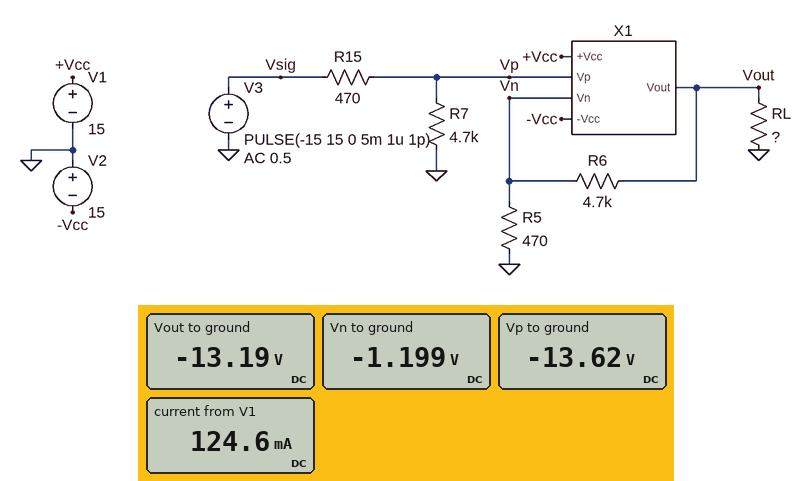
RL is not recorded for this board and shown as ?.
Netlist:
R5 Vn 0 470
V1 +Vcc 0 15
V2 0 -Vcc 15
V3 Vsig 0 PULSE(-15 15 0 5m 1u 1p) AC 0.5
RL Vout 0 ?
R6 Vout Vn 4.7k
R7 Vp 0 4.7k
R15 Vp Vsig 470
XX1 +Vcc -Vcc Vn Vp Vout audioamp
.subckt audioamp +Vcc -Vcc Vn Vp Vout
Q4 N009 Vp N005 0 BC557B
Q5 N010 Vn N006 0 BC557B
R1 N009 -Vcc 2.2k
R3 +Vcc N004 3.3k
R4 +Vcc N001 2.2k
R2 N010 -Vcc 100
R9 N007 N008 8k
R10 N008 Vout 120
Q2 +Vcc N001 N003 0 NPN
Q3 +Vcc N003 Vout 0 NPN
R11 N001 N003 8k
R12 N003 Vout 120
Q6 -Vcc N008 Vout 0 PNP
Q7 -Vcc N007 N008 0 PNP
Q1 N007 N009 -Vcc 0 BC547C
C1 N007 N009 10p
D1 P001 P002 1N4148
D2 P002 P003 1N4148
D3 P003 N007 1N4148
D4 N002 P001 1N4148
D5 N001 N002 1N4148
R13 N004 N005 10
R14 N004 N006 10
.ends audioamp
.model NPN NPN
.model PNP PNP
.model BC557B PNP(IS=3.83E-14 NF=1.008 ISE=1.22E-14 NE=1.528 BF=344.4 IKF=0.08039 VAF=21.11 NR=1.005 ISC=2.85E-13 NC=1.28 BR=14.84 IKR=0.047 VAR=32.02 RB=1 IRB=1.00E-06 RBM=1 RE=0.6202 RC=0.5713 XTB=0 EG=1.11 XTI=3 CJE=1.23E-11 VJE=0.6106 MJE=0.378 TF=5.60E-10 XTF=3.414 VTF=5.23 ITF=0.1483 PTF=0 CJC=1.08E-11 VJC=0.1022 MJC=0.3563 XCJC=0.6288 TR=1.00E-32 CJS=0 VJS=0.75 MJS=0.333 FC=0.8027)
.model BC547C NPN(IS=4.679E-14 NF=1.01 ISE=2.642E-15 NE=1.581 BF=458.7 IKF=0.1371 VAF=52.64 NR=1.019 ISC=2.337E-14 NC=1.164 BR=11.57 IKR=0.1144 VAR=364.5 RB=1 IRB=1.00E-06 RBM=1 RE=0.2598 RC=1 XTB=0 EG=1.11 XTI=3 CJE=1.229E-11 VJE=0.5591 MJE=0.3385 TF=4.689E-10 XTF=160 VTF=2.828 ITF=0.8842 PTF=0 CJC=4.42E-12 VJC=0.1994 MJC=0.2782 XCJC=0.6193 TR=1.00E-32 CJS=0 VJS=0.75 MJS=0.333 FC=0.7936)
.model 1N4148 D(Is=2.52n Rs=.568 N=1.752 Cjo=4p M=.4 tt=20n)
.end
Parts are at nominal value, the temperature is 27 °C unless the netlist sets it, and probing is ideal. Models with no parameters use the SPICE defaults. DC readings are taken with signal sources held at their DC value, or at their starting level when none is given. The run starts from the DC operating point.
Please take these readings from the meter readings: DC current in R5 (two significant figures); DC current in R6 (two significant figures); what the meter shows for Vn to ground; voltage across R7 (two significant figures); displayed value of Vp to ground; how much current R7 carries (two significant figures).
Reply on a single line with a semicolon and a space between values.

2.6 mA; 2.6 mA; -1.199 V; 14 V; -13.62 V; 2.9 mA
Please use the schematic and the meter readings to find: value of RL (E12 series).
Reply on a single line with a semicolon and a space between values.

18 Ω
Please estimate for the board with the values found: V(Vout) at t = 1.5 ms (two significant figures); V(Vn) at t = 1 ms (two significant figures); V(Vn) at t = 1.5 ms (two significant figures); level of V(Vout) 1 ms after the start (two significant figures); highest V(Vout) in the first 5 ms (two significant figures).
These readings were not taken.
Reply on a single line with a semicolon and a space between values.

-13 V; -1.2 V; -1.2 V; -13 V; 13 V
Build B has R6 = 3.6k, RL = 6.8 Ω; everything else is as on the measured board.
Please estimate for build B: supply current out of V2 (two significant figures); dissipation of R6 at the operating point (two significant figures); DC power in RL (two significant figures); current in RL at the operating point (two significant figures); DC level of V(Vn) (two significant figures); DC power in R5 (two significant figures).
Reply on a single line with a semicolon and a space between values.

2.0 A; 38 mW; 25 W; 1.9 A; -1.5 V; 4.9 mW
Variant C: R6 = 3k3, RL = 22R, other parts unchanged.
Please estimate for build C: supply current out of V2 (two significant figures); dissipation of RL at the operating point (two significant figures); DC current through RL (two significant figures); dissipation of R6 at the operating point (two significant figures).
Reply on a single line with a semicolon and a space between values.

750 mA; 7.9 W; 600 mA; 40 mW
